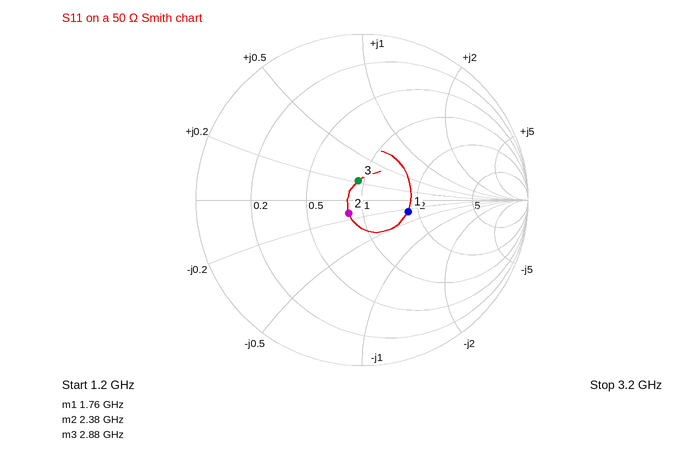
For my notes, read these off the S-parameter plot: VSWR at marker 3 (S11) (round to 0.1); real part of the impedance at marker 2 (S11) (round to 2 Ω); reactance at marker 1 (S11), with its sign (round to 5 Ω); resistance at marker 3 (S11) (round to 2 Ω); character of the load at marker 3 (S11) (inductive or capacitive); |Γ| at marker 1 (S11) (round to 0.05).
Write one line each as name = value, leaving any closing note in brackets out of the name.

VSWR at marker 3 (S11) = 1.3
real part of the impedance at marker 2 (S11) = 42 Ω
reactance at marker 1 (S11), with its sign = -15 Ω
resistance at marker 3 (S11) = 46 Ω
character of the load at marker 3 (S11) = inductive
|Γ| at marker 1 (S11) = 0.30
